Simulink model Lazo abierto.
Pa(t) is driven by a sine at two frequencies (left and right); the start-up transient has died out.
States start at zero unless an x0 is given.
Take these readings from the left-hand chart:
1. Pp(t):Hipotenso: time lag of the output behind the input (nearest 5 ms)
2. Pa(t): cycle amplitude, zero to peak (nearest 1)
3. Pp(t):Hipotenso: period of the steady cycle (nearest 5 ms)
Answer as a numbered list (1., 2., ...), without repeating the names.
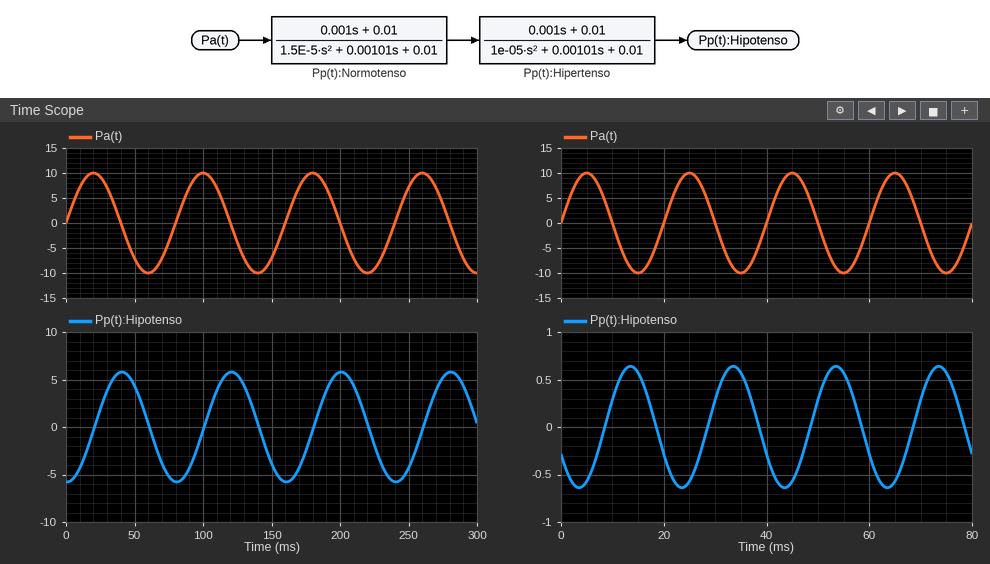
1. 20 ms
2. 10
3. 80 ms
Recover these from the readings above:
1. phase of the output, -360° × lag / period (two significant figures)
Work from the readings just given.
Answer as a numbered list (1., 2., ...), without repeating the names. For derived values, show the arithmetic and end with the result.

1. -360 × 20 / 80 = -90°
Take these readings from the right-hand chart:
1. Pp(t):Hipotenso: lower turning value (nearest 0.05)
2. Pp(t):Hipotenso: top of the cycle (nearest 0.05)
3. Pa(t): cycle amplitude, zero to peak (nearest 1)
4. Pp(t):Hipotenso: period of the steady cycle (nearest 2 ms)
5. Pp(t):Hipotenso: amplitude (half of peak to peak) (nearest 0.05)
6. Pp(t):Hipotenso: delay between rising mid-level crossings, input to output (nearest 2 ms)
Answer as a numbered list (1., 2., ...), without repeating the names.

1. -0.65
2. 0.65
3. 10
4. 20 ms
5. 0.65
6. 8 ms
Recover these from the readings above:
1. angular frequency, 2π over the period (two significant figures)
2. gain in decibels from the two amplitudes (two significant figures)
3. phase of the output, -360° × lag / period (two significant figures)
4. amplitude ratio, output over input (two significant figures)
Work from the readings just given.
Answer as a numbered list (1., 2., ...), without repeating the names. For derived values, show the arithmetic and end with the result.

1. 2π / 20 = 0.31 rad/ms
2. 20 log10(0.65 / 10) = -24 dB
3. -360 × 8 / 20 = -140°
4. 0.65 / 10 = 0.065
